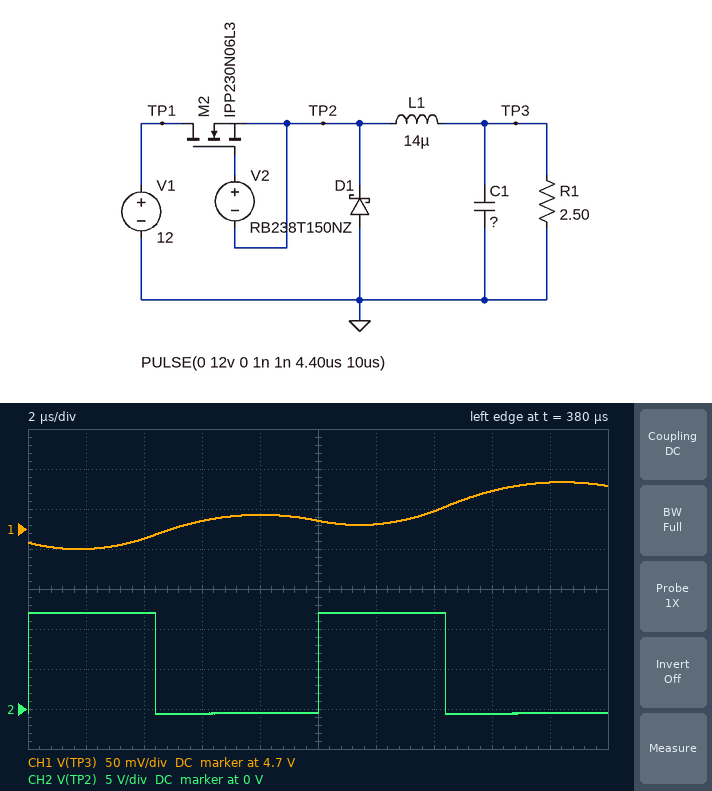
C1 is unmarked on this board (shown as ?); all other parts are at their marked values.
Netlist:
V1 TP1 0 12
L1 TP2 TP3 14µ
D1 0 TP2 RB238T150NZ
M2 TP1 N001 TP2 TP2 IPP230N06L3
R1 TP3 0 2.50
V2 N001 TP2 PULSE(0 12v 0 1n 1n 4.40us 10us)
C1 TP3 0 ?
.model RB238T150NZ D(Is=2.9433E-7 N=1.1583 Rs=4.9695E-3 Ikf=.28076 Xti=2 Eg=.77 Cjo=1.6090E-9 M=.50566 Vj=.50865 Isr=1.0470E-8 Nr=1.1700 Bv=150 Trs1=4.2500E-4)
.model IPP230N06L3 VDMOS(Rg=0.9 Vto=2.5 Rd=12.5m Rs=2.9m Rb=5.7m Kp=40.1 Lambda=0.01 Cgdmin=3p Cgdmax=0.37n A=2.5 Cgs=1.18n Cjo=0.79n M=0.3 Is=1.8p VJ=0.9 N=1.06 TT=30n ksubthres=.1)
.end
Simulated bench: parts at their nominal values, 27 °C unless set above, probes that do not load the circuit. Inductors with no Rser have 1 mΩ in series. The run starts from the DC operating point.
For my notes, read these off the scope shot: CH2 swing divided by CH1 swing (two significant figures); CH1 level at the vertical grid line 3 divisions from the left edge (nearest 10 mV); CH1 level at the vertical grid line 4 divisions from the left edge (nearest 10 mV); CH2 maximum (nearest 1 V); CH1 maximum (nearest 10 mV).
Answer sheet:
150
4.71 V
4.72 V
12 V
4.76 V
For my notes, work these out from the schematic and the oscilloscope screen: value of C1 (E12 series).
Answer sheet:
100 µF
